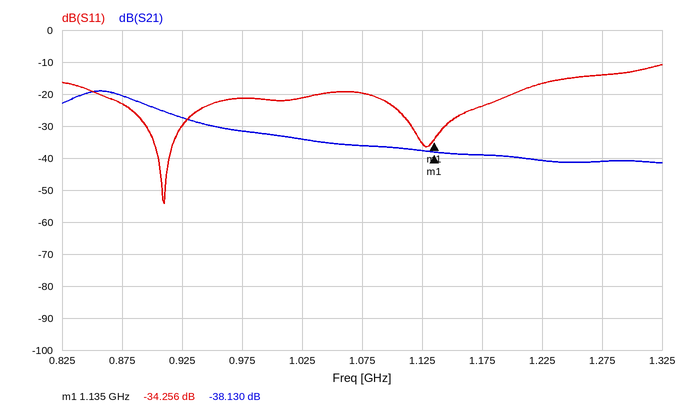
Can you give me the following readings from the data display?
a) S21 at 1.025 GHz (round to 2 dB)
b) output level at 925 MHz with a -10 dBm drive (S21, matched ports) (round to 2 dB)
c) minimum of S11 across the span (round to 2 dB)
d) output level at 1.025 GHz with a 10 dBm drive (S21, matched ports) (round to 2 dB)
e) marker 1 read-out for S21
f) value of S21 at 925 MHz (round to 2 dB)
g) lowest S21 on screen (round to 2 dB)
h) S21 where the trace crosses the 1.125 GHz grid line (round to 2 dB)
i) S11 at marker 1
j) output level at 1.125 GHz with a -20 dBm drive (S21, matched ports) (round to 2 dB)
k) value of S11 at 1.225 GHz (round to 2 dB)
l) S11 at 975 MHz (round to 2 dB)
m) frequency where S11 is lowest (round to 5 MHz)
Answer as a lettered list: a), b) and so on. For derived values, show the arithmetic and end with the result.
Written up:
a) -34 dB
b) -10 dBm + (-28 dB) = -38 dBm
c) -54 dB
d) 10 dBm + (-34 dB) = -24 dBm
e) -38.130 dB
f) -28 dB
g) -42 dB
h) -38 dB
i) -34.256 dB
j) -20 dBm + (-38 dB) = -58 dBm
k) -16 dB
l) -22 dB
m) 910 MHz
